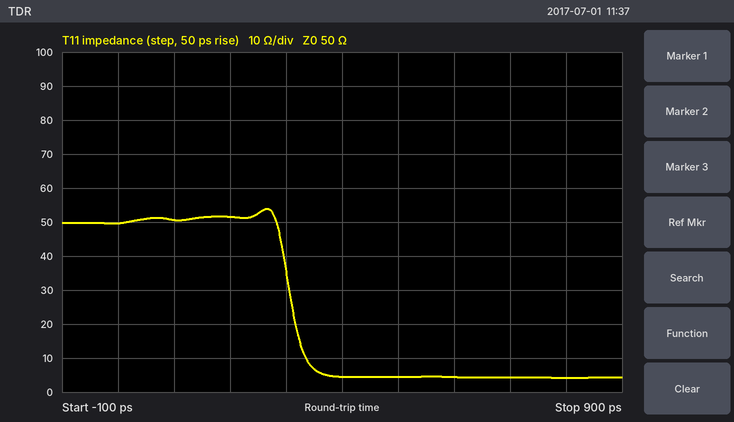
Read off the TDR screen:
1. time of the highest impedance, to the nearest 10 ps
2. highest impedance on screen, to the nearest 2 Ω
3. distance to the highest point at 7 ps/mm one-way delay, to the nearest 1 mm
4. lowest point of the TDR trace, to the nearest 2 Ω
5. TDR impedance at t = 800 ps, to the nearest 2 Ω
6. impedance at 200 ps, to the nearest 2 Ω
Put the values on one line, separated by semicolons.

270 ps; 54 Ω; 19 mm; 4 Ω; 4 Ω; 52 Ω
